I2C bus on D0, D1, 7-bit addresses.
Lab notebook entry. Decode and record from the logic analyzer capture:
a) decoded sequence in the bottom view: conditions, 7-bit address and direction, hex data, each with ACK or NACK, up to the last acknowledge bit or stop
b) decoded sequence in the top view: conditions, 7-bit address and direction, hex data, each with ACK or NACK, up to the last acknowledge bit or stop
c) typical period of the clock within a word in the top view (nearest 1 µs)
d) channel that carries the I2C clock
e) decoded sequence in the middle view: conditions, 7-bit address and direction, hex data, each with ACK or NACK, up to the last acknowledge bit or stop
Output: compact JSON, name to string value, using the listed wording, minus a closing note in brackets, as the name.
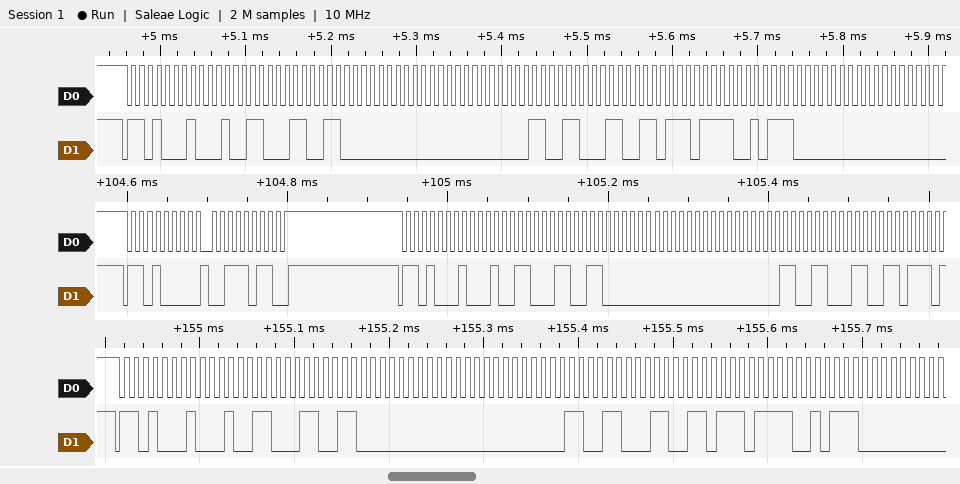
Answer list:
{"decoded sequence in the bottom view: conditions, 7-bit address and direction, hex data, each with ACK or NACK, up to the last acknowledge bit or stop": "start, address 68 read ACK, 26 ACK, 66 ACK, 00 ACK, 00 ACK, 33 ACK, 33 ACK, EF ACK, 5C ACK", "decoded sequence in the top view: conditions, 7-bit address and direction, hex data, each with ACK or NACK, up to the last acknowledge bit or stop": "start, address 68 read ACK, 26 ACK, 66 ACK, 00 ACK, 00 ACK, 33 ACK, 33 ACK, EF ACK, 5C ACK, 00 ACK", "typical period of the clock within a word in the top view": "10 µs", "channel that carries the I2C clock": "D0", "decoded sequence in the middle view: conditions, 7-bit address and direction, hex data, each with ACK or NACK, up to the last acknowledge bit or stop": "start, address 68 write ACK, 3B ACK, stop, start, address 68 read ACK, 26 ACK, 66 ACK, 00 ACK, 00 ACK, 33 ACK, 33 ACK"}
